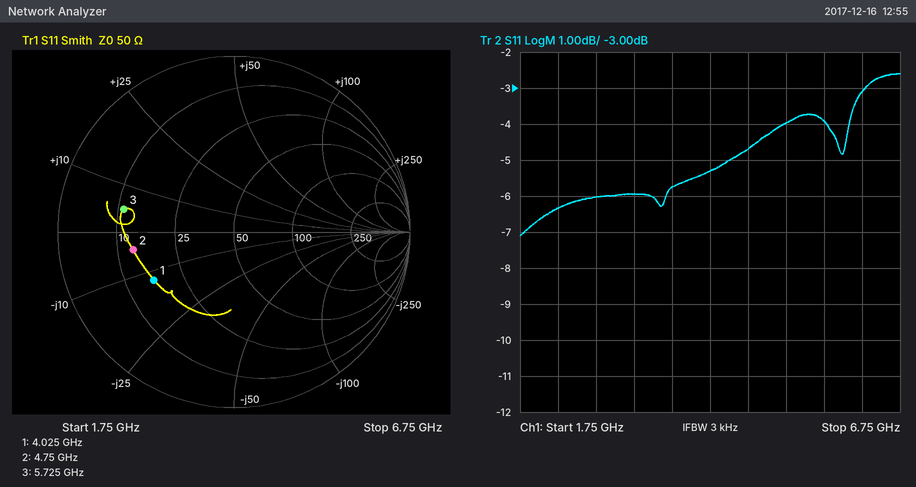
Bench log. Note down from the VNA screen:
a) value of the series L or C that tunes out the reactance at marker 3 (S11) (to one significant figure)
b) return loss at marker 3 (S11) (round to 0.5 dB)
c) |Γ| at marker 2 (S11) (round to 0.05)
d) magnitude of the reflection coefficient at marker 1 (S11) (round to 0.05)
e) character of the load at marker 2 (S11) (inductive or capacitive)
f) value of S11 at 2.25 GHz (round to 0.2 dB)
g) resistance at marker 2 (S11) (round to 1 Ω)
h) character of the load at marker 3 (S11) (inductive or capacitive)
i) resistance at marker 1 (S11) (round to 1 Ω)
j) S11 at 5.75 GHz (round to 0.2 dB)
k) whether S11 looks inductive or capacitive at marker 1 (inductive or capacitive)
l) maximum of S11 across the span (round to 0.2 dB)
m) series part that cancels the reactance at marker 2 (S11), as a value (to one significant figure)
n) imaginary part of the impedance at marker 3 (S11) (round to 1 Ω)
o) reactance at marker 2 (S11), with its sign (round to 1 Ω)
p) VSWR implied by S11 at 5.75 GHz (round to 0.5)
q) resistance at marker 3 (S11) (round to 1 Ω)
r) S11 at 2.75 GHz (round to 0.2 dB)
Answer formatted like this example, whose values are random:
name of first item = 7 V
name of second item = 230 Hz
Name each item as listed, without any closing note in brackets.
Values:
value of the series L or C that tunes out the reactance at marker 3 (S11) = 6 pF
return loss at marker 3 (S11) = 4.0 dB
|Γ| at marker 2 (S11) = 0.60
magnitude of the reflection coefficient at marker 1 (S11) = 0.55
character of the load at marker 2 (S11) = capacitive
value of S11 at 2.25 GHz = -6.4 dB
resistance at marker 2 (S11) = 13 Ω
character of the load at marker 3 (S11) = inductive
resistance at marker 1 (S11) = 16 Ω
S11 at 5.75 GHz = -4.0 dB
whether S11 looks inductive or capacitive at marker 1 = capacitive
maximum of S11 across the span = -2.6 dB
series part that cancels the reactance at marker 2 (S11), as a value = 100 pH
imaginary part of the impedance at marker 3 (S11) = +5 Ω
reactance at marker 2 (S11), with its sign = -4 Ω
VSWR implied by S11 at 5.75 GHz = 4.5
resistance at marker 3 (S11) = 11 Ω
S11 at 2.75 GHz = -6.0 dB
